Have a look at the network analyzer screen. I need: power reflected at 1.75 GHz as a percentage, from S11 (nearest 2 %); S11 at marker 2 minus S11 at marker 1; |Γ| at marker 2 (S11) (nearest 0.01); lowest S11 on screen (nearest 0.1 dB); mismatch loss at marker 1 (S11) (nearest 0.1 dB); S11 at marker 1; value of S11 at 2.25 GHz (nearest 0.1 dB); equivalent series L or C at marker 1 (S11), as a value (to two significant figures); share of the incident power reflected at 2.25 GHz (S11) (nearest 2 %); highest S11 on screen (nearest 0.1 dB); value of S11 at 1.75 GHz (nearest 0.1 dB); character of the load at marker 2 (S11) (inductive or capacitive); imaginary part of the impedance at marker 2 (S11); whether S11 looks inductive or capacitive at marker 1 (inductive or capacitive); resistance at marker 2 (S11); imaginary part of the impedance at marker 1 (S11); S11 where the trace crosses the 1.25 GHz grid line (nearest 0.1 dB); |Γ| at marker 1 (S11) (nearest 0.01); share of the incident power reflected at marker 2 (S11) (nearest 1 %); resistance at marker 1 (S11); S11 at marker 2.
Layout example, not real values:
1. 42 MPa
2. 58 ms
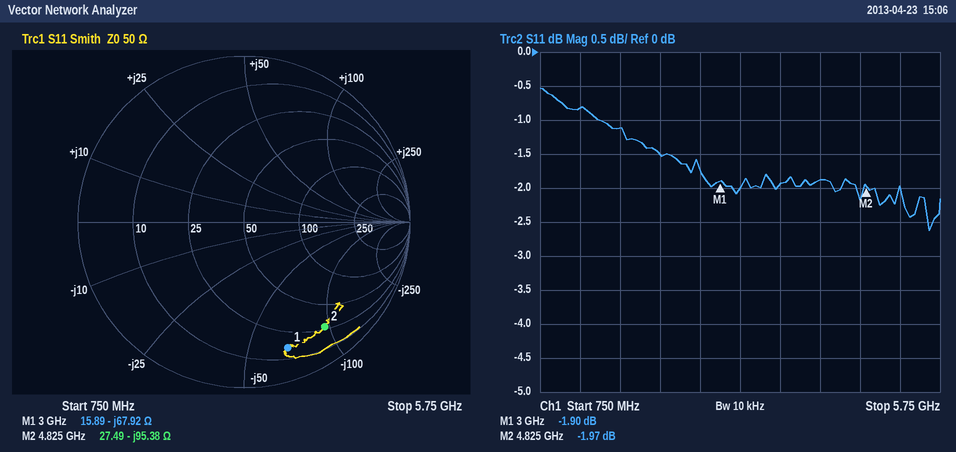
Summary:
1. 78 %
2. -0.07 dB
3. 0.80
4. -2.6 dB
5. 4.5 dB
6. -1.90 dB
7. -1.5 dB
8. 780 fF
9. 70 %
10. -0.5 dB
11. -1.1 dB
12. capacitive
13. -95.38 Ω
14. capacitive
15. 27.49 Ω
16. -67.92 Ω
17. -0.8 dB
18. 0.80
19. 64 %
20. 15.89 Ω
21. -1.97 dB
